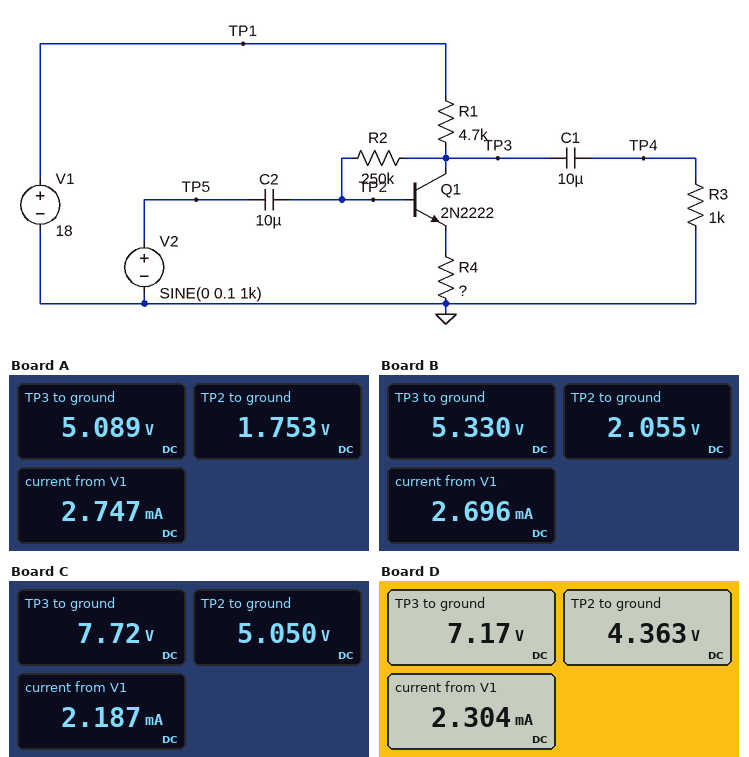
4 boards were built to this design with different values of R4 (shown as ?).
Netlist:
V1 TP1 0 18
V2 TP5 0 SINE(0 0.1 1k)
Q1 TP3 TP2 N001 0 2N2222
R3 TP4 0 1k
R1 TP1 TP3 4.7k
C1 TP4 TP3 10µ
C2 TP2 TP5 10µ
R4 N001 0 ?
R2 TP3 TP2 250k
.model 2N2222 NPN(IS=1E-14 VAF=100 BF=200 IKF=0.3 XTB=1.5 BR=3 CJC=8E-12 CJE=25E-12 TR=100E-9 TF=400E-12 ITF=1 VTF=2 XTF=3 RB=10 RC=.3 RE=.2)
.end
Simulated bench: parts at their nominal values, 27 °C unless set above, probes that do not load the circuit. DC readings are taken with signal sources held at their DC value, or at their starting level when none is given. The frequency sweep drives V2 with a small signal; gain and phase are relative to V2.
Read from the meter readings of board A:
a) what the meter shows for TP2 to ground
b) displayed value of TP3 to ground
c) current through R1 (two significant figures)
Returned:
1.753 V
5.089 V
2.7 mA
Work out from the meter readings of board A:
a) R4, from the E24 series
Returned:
390 Ω
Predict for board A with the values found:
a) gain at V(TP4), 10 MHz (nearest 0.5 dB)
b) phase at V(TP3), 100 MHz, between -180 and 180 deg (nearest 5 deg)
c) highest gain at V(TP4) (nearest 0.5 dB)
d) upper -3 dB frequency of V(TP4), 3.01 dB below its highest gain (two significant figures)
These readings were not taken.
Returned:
6.0 dB
50 deg
6.0 dB
74 MHz
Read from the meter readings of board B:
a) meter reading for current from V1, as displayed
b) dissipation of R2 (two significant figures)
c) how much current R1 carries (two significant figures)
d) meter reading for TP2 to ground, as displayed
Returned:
2.696 mA
43 µW
2.7 mA
2.055 V
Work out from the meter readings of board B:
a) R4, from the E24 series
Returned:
510 Ω
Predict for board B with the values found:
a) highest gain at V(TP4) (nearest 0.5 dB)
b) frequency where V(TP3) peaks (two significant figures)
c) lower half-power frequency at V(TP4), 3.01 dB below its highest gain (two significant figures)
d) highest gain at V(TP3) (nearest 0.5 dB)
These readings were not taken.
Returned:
4.0 dB
1.5 Hz
2.5 Hz
18.0 dB
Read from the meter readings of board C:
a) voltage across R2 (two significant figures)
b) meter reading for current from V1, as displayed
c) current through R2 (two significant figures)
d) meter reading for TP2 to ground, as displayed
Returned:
2.7 V
2.187 mA
11 µA
5.050 V
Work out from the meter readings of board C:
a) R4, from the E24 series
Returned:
2 kΩ
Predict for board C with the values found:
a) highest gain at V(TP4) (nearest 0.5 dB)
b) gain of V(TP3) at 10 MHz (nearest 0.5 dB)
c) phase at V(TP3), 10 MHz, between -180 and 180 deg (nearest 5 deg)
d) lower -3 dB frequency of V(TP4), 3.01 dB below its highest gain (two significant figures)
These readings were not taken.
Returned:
0 dB
-6.5 dB
130 deg
29 MHz
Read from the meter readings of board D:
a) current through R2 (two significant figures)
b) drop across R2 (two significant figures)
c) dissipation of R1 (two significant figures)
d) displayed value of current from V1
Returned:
11 µA
2.8 V
25 mW
2.304 mA
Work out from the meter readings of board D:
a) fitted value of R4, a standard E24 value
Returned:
1.6 kΩ
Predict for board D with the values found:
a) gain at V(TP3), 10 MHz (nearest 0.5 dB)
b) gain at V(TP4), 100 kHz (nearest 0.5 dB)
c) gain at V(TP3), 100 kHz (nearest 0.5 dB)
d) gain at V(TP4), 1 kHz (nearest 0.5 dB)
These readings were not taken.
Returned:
-5.0 dB
-6.0 dB
-6.0 dB
-6.0 dB
